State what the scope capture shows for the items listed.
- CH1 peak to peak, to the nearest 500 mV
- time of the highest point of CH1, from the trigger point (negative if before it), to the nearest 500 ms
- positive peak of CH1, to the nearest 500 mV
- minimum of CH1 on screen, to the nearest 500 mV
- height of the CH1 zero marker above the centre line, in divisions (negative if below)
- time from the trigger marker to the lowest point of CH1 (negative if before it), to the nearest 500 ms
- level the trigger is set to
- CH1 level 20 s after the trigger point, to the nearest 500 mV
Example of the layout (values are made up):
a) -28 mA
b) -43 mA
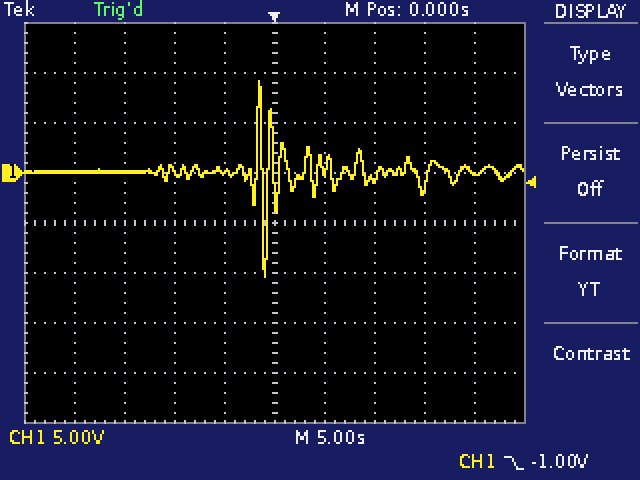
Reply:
a) 19.5 V
b) -1.5 s
c) 9.0 V
d) -10.5 V
e) +1.0 div
f) -1.0 s
g) -1.00 V
h) 0.0 V
